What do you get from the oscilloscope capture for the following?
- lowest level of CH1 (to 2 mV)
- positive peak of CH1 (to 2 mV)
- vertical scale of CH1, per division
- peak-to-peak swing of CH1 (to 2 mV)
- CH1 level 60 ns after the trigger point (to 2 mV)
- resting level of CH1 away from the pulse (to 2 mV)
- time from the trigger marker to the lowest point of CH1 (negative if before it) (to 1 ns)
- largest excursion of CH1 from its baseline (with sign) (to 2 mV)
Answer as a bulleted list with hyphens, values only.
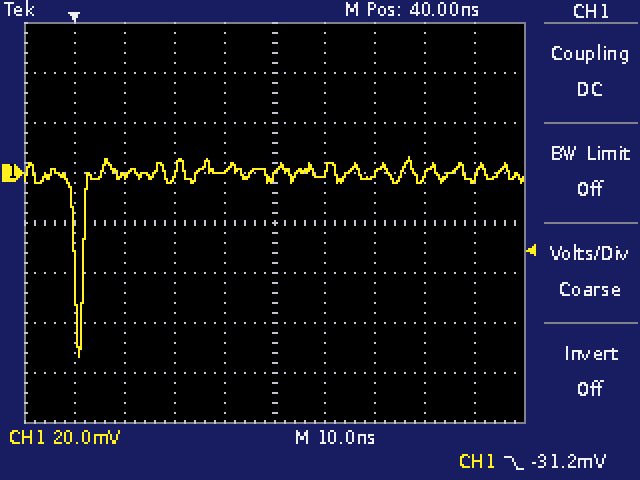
- -74 mV
- 6 mV
- 20 mV
- 80 mV
- 0 mV
- 0 mV
- +1 ns
- -74 mV
